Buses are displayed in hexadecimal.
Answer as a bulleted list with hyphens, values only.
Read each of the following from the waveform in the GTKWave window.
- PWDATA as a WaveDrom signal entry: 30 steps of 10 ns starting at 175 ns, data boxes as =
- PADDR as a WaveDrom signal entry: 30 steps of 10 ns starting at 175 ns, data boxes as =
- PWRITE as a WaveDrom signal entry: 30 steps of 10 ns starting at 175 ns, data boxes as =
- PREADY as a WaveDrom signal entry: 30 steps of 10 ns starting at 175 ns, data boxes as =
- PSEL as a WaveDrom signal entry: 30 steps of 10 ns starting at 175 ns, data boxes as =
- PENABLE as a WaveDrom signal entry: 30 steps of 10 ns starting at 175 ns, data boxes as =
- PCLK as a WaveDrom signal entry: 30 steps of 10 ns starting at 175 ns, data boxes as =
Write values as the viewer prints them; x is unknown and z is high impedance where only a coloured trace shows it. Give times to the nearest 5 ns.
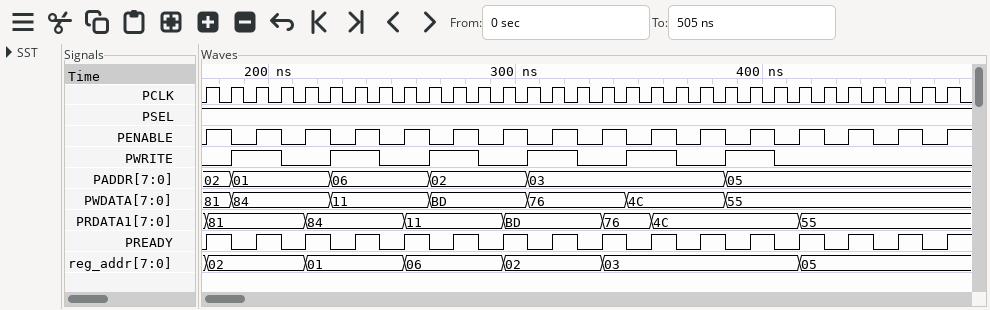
- {name: 'PWDATA', wave: '==...=...=...=...=...=........', data: '81 84 11 BD 76 4C 55'}
- {name: 'PADDR', wave: '==...=...=...=.......=........', data: '02 01 06 02 03 05'}
- {name: 'PWRITE', wave: '01.0.1.0.1.0.1.0.1.0.1.0......'}
- {name: 'PREADY', wave: '101010101010101010101010101010'}
- {name: 'PSEL', wave: '1.............................'}
- {name: 'PENABLE', wave: '101010101010101010101010101010'}
- {name: 'PCLK', wave: 'p.............................'}
